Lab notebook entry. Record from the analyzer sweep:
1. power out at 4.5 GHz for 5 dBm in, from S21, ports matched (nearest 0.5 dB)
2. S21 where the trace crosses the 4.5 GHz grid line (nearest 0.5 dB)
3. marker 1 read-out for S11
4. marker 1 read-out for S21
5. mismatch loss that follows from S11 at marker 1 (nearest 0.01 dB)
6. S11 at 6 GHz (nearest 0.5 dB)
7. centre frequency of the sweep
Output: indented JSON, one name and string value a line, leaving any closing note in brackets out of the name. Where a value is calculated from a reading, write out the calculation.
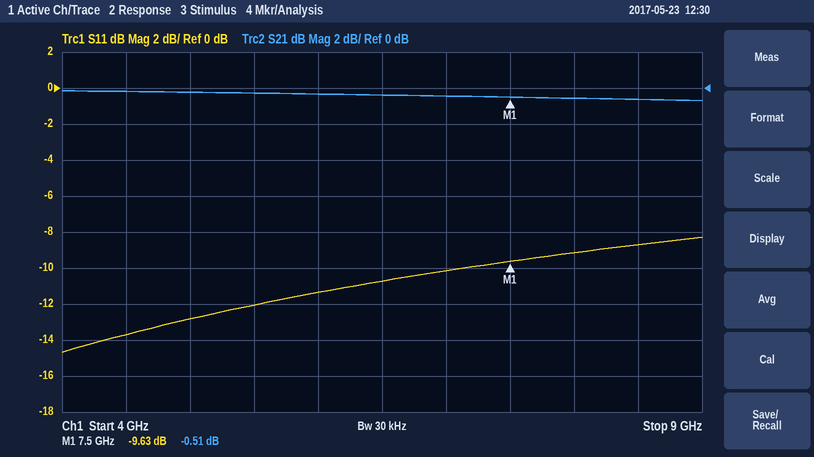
{
  "power out at 4.5 GHz for 5 dBm in, from S21, ports matched": "5 dBm + (0.0 dB) = 5.0 dBm",
  "S21 where the trace crosses the 4.5 GHz grid line": "0.0 dB",
  "marker 1 read-out for S11": "-9.63 dB",
  "marker 1 read-out for S21": "-0.51 dB",
  "mismatch loss that follows from S11 at marker 1": "−10 log10(1 − 10^(-9.63/10)) ≈ 0.50 dB",
  "S11 at 6 GHz": "-11.5 dB",
  "centre frequency of the sweep": "6.5 GHz"
}
